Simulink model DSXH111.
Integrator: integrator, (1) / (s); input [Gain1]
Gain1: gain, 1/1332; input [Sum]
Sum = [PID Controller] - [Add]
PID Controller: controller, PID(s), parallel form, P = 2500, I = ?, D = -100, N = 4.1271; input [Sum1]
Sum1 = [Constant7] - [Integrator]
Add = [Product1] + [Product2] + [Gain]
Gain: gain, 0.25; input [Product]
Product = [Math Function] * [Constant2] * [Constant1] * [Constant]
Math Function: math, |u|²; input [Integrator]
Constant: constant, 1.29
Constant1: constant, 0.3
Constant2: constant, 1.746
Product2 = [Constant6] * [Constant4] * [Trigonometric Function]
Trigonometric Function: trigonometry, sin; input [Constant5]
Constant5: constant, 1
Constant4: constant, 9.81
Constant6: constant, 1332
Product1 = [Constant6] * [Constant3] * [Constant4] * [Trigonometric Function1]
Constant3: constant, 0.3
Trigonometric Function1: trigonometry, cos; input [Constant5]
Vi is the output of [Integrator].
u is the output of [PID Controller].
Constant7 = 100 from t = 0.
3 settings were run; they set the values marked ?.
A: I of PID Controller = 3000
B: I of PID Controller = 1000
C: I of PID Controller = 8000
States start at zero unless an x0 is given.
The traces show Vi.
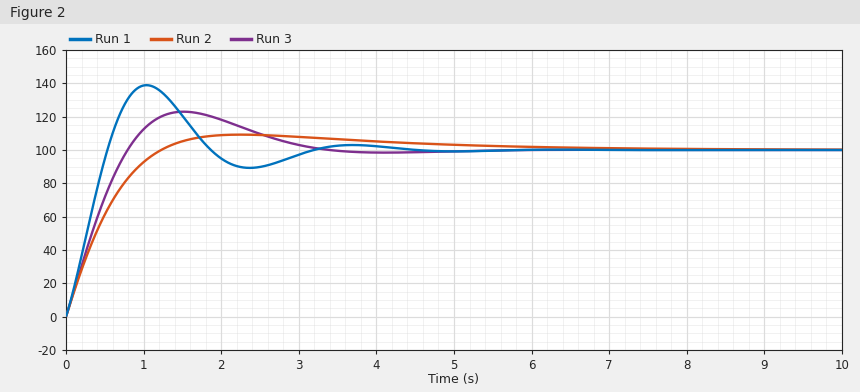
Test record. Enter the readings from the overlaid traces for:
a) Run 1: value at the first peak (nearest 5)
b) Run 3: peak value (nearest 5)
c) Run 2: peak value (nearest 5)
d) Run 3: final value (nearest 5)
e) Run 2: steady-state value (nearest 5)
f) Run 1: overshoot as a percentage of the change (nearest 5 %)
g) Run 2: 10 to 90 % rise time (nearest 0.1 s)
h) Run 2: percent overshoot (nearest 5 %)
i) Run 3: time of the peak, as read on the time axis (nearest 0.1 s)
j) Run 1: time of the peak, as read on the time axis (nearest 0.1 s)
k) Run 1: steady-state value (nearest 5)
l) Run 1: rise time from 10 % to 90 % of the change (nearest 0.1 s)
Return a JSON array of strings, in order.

["140", "125", "110", "100", "100", "40 %", "0.9 s", "10 %", "1.5 s", "1.0 s", "100", "0.4 s"]
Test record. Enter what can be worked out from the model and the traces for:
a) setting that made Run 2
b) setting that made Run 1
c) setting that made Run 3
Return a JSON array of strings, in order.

["B", "C", "A"]
